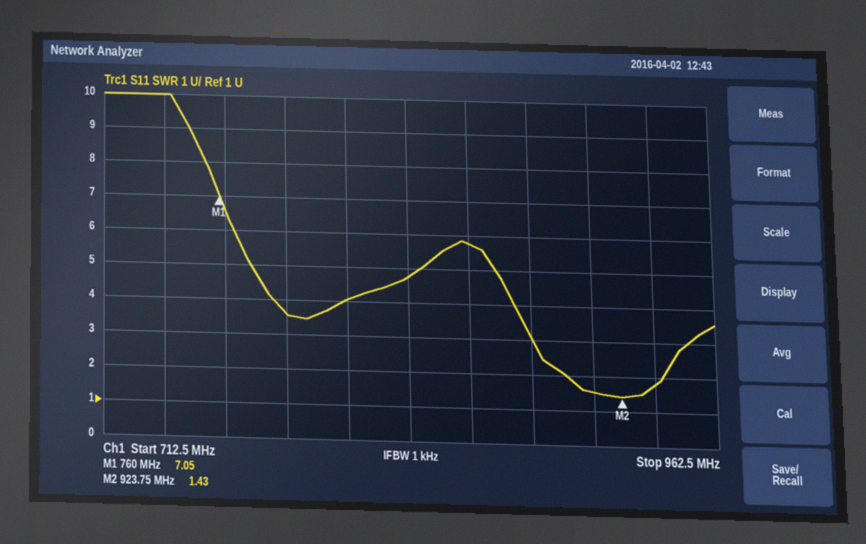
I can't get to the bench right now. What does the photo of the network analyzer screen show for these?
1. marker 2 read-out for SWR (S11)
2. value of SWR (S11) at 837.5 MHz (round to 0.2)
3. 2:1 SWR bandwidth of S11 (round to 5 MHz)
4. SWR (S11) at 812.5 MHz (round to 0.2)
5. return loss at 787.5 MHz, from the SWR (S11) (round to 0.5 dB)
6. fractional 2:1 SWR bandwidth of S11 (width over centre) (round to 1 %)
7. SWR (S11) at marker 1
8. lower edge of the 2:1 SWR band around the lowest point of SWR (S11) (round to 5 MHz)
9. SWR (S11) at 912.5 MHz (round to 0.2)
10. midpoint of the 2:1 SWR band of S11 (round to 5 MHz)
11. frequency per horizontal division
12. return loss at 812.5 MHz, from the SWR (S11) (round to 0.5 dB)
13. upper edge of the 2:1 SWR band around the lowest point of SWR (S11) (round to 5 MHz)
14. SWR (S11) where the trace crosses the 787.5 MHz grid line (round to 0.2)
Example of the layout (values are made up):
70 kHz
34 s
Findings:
1.43
4.8
40 MHz
4.0
5.0 dB
4 %
7.05
900 MHz
1.6
920 MHz
25 MHz
4.5 dB
940 MHz
3.6
